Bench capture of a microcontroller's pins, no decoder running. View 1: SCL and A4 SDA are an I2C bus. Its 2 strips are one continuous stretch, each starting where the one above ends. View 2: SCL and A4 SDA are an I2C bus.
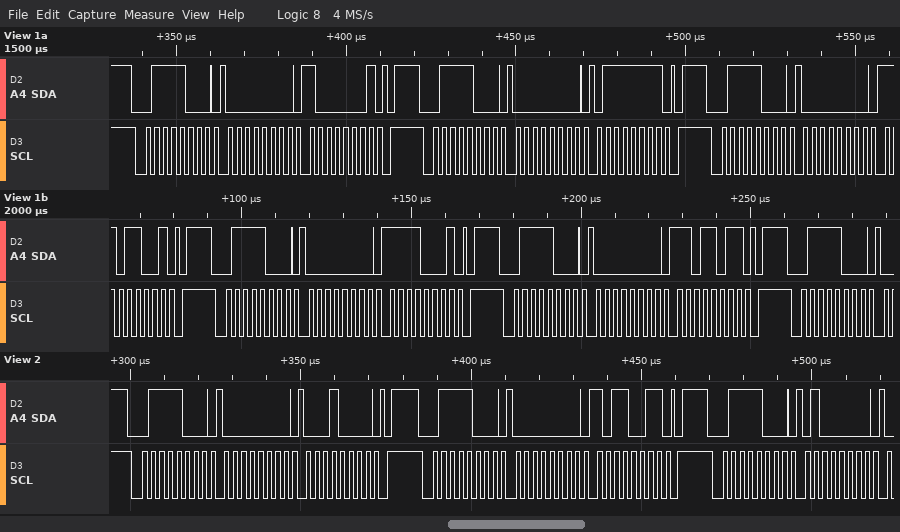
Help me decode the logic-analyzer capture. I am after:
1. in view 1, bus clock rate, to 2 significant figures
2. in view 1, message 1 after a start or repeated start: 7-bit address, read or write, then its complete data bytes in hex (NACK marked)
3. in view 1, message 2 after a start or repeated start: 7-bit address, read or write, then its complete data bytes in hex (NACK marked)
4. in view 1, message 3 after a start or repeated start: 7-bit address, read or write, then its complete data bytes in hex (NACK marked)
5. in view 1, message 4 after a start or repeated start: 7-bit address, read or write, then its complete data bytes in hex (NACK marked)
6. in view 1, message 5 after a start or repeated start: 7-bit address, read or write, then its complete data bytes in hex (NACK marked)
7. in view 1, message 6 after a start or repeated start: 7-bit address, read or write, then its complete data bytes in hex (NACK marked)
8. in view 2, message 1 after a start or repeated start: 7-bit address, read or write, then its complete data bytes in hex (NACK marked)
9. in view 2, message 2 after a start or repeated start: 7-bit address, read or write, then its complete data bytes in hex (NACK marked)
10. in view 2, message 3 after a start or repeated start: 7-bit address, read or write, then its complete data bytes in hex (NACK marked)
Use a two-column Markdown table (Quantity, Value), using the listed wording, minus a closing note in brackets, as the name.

| Quantity | Value |
|---|---|
| in view 1, bus clock rate, to 2 significant figures | 400 kHz |
| in view 1, message 1 after a start or repeated start: 7-bit address, read or write, then its complete data bytes in hex | 0x3C write: 00 81 |
| in view 1, message 2 after a start or repeated start: 7-bit address, read or write, then its complete data bytes in hex | 0x3C write: 00 7F |
| in view 1, message 3 after a start or repeated start: 7-bit address, read or write, then its complete data bytes in hex | 0x3C write: 00 D9 |
| in view 1, message 4 after a start or repeated start: 7-bit address, read or write, then its complete data bytes in hex | 0x3C write: 00 F1 |
| in view 1, message 5 after a start or repeated start: 7-bit address, read or write, then its complete data bytes in hex | 0x3C write: 00 DB |
| in view 1, message 6 after a start or repeated start: 7-bit address, read or write, then its complete data bytes in hex | 0x3C write |
| in view 2, message 1 after a start or repeated start: 7-bit address, read or write, then its complete data bytes in hex | 0x3C write: 00 10 |
| in view 2, message 2 after a start or repeated start: 7-bit address, read or write, then its complete data bytes in hex | 0x3C write: 00 B3 |
| in view 2, message 3 after a start or repeated start: 7-bit address, read or write, then its complete data bytes in hex | 0x3C write: 40 |
